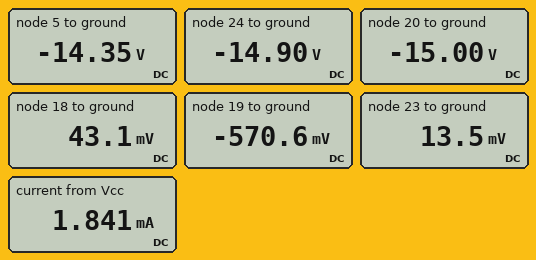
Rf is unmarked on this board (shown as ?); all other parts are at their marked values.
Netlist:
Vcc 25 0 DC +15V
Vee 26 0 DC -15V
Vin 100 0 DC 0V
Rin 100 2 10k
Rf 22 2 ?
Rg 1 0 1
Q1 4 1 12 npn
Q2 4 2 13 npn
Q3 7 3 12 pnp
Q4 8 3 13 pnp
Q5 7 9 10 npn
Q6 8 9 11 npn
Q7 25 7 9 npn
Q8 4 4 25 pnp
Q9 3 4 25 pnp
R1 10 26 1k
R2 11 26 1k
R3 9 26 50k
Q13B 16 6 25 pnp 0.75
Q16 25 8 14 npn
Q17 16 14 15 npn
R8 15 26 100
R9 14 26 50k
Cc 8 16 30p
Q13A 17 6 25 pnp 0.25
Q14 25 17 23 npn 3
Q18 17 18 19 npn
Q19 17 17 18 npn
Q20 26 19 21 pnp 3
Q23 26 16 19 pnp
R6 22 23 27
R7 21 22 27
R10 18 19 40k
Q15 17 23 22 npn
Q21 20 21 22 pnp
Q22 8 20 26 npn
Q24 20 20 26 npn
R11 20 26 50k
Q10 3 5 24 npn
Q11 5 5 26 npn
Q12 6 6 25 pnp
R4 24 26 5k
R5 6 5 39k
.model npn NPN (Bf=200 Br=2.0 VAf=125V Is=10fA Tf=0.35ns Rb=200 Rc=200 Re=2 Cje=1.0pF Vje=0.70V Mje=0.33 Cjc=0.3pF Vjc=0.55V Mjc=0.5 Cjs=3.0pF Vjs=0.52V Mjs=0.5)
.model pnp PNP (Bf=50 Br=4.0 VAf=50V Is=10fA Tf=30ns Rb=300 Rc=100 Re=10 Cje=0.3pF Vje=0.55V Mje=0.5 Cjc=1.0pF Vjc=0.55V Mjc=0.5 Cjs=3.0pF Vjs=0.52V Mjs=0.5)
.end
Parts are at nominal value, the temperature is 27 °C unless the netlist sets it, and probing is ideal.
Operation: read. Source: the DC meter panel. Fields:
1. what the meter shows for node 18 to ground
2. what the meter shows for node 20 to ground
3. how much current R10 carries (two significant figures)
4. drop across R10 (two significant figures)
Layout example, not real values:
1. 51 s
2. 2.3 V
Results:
1. 43.1 mV
2. -15.00 V
3. 15 µA
4. 610 mV
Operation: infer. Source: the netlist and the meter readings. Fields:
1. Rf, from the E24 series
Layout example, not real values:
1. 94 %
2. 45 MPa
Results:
1. 130 kΩ
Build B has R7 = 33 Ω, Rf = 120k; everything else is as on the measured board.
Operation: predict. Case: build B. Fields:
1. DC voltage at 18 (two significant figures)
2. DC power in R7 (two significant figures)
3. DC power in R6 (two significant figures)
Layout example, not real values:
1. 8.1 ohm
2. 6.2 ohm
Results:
1. 42 mV
2. 930 nW
3. 760 nW
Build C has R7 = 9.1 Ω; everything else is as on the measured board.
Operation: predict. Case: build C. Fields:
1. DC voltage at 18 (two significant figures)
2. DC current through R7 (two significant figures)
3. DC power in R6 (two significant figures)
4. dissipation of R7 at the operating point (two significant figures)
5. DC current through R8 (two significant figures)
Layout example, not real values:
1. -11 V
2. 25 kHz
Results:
1. 45 mV
2. 180 µA
3. 870 nW
4. 290 nW
5. 660 µA
